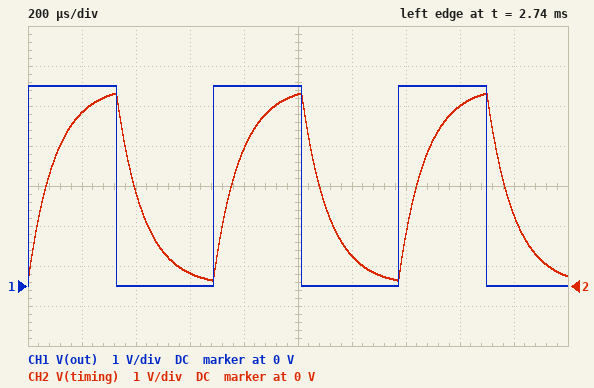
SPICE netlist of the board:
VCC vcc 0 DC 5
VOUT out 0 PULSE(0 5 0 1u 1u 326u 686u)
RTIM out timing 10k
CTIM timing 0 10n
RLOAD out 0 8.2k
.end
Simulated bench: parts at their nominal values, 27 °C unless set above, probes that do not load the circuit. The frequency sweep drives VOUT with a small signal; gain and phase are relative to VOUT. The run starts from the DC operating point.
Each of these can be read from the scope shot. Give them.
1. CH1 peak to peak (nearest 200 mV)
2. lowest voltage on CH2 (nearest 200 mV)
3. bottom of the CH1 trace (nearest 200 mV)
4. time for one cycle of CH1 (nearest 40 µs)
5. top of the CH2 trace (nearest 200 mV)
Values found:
5.0 V
200 mV
0 V
680 µs
4.8 V
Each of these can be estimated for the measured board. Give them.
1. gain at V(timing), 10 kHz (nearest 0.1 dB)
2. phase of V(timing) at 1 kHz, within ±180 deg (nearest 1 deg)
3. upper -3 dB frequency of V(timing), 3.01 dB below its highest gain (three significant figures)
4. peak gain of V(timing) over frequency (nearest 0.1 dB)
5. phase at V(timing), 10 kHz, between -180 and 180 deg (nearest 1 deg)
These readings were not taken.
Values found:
-16.1 dB
-32 deg
1.59 kHz
0 dB
-81 deg
